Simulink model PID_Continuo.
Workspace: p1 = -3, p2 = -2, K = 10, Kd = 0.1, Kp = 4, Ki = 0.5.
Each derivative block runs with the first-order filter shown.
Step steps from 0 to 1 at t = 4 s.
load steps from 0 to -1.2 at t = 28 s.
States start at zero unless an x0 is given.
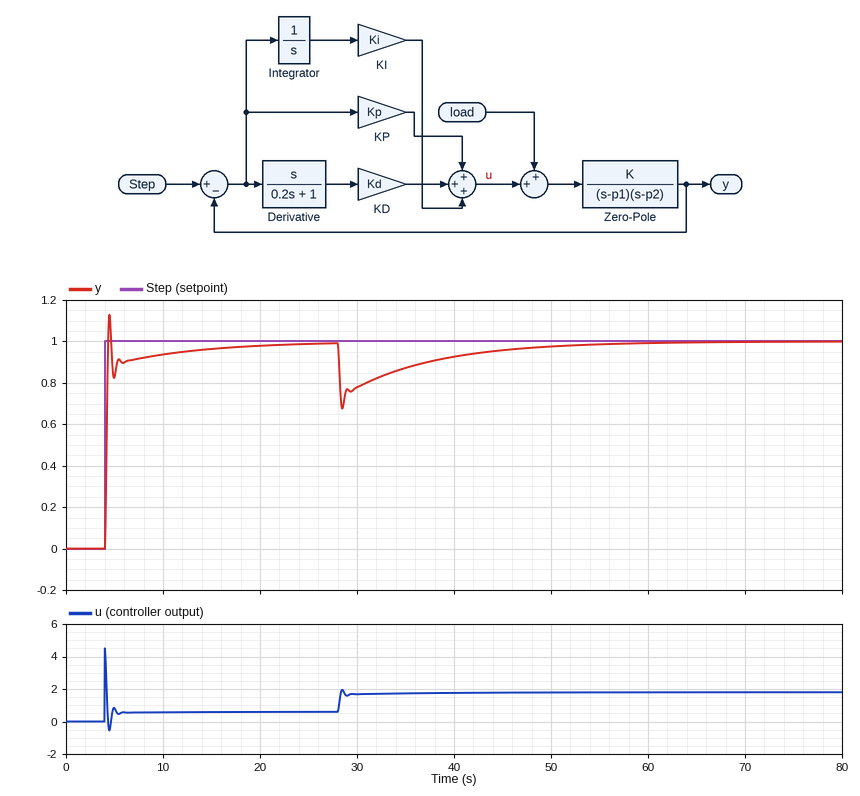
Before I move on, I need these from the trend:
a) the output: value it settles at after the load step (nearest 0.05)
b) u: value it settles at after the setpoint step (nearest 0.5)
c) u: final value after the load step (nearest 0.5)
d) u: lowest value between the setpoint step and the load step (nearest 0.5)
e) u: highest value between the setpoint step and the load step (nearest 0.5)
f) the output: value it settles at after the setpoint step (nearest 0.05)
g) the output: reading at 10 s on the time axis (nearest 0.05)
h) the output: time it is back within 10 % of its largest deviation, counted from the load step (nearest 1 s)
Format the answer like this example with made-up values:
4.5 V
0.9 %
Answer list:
1.00
0.5
2.0
-0.5
4.5
1.00
0.95
20 s
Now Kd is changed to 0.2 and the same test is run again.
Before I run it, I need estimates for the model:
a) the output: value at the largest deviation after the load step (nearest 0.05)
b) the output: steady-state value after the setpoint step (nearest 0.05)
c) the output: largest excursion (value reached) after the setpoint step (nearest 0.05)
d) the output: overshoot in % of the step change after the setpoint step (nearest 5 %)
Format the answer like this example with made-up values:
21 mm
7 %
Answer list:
0.70
1.00
1.10
10 %
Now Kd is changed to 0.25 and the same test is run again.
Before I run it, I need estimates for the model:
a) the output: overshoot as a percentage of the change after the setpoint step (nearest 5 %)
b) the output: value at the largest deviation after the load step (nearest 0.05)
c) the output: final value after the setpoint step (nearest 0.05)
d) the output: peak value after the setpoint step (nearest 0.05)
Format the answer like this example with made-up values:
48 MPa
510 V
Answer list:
10 %
0.70
1.00
1.10
